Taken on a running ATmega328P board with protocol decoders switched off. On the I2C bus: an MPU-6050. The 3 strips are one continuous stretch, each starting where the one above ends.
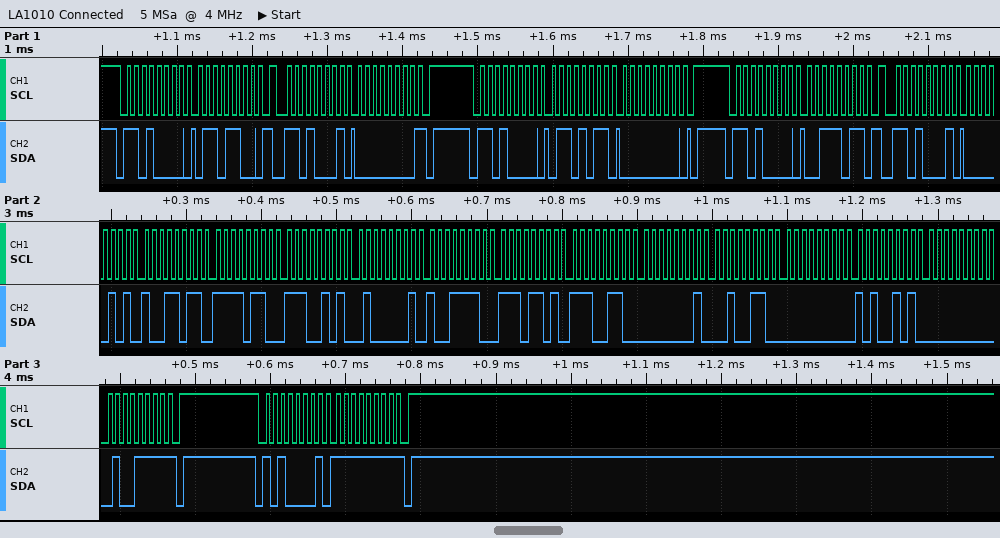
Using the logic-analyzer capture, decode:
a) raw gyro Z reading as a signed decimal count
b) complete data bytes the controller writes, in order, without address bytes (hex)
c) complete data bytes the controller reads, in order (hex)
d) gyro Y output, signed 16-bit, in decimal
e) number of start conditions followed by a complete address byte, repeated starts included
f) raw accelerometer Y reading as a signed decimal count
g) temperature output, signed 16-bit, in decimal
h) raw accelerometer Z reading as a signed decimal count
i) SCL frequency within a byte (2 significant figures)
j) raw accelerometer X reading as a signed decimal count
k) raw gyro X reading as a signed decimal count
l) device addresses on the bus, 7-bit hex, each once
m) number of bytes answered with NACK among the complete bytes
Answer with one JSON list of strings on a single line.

["79", "6C 6B 00 3B", "00 05 9B F6 E5 41 9E ED E6 01 26 00 A5 00 4F FF", "165", "6", "-2331", "-4634", "16798", "100 kHz", "1435", "294", "0x68 0x50", "3"]
